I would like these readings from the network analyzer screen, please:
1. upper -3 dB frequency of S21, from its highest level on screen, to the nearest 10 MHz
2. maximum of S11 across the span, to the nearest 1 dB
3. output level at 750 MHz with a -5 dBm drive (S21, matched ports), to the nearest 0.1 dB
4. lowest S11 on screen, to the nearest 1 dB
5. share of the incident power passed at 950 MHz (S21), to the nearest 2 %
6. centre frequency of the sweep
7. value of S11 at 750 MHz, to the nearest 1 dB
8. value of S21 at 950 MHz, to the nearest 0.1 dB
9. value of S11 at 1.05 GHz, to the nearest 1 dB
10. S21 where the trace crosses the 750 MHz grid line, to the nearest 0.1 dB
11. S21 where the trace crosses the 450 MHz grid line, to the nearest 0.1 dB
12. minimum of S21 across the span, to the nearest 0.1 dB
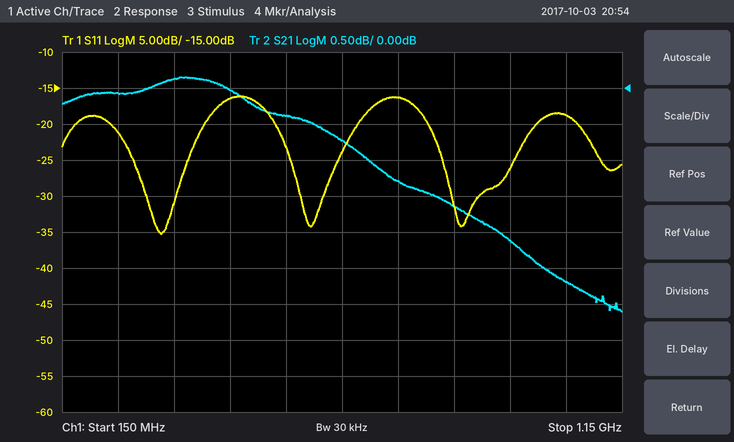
1.09 GHz
-16 dB
-6.3 dBm
-35 dB
62 %
650 MHz
-16 dB
-2.1 dB
-19 dB
-1.3 dB
0.0 dB
-3.1 dB
